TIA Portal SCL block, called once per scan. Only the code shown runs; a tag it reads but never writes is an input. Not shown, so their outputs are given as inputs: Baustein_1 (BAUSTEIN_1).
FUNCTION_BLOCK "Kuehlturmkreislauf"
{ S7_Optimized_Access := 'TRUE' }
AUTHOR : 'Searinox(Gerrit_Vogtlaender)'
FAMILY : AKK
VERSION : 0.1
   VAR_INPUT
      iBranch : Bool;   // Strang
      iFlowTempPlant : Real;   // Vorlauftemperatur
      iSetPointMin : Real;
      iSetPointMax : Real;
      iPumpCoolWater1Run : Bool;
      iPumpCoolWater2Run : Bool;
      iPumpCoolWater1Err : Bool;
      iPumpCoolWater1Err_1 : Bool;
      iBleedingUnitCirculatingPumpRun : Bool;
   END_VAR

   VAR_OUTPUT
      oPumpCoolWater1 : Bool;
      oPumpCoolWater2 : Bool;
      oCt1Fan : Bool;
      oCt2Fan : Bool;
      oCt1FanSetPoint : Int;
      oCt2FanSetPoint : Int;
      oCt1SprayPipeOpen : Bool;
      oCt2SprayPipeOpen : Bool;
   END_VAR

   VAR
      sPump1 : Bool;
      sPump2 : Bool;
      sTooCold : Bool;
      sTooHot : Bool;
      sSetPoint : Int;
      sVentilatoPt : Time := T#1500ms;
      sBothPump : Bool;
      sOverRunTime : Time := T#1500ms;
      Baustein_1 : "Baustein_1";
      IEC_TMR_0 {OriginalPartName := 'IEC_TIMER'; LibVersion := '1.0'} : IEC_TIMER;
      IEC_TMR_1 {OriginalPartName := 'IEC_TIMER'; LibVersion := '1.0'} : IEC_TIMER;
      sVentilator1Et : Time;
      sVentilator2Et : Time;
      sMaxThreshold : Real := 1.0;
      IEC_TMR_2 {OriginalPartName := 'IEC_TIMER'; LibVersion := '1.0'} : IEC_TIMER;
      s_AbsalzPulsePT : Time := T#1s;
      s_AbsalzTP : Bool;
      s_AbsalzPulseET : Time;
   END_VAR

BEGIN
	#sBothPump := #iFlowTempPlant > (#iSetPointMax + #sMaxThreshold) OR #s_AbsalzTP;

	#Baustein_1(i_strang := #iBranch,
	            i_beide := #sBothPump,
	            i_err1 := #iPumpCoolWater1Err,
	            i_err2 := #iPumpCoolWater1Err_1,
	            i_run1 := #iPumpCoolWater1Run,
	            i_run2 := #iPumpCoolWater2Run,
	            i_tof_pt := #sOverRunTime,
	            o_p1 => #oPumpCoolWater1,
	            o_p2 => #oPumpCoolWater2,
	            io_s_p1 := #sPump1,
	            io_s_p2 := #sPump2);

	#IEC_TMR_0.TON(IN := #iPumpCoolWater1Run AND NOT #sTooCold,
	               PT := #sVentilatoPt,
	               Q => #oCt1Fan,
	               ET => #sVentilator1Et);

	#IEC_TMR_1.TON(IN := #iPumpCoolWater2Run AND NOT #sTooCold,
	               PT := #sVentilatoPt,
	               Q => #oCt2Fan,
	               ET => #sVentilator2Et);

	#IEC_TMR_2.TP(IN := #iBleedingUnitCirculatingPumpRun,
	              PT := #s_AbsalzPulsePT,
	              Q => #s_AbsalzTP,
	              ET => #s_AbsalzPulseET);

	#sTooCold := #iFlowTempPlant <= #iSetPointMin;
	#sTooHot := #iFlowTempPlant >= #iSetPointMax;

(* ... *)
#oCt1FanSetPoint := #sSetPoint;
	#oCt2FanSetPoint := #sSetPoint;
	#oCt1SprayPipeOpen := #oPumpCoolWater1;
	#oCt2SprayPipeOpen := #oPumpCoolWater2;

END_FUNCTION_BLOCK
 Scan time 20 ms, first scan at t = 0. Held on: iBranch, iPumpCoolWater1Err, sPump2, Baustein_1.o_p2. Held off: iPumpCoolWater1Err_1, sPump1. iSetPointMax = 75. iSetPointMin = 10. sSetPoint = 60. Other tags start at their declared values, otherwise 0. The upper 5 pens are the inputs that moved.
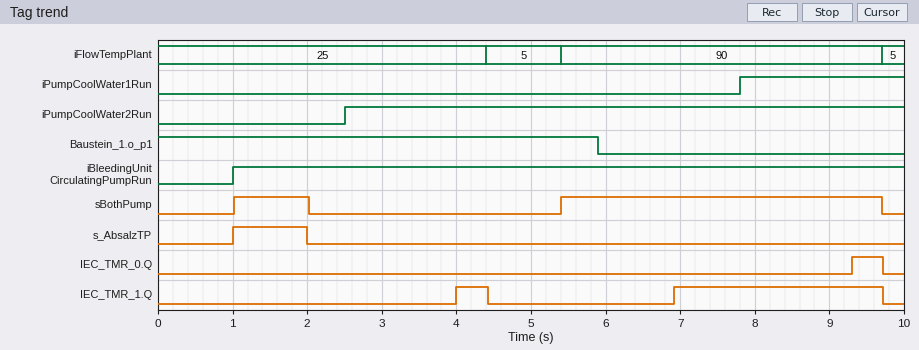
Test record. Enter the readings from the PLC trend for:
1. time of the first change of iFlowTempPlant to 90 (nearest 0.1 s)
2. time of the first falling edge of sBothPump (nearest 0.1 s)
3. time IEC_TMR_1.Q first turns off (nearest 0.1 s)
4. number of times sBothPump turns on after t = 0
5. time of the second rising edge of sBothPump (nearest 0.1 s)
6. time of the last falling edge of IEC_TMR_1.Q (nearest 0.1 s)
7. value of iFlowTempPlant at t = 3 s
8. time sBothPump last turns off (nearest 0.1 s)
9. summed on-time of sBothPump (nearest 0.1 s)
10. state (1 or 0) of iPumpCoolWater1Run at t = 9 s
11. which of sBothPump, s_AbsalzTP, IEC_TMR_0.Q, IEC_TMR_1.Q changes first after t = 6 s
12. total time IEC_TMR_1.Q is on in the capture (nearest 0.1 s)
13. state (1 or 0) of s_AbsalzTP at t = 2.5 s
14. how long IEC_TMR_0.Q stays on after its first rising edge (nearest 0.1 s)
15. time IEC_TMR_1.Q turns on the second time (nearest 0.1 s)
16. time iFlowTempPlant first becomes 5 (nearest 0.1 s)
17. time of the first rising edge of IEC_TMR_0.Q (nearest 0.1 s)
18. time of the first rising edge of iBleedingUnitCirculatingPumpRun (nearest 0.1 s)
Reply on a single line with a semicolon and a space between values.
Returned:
5.4 s; 2.0 s; 4.4 s; 2; 5.4 s; 9.7 s; 25; 9.7 s; 5.3 s; 1; IEC_TMR_1.Q; 3.2 s; 0; 0.4 s; 6.9 s; 4.4 s; 9.3 s; 1.0 s
